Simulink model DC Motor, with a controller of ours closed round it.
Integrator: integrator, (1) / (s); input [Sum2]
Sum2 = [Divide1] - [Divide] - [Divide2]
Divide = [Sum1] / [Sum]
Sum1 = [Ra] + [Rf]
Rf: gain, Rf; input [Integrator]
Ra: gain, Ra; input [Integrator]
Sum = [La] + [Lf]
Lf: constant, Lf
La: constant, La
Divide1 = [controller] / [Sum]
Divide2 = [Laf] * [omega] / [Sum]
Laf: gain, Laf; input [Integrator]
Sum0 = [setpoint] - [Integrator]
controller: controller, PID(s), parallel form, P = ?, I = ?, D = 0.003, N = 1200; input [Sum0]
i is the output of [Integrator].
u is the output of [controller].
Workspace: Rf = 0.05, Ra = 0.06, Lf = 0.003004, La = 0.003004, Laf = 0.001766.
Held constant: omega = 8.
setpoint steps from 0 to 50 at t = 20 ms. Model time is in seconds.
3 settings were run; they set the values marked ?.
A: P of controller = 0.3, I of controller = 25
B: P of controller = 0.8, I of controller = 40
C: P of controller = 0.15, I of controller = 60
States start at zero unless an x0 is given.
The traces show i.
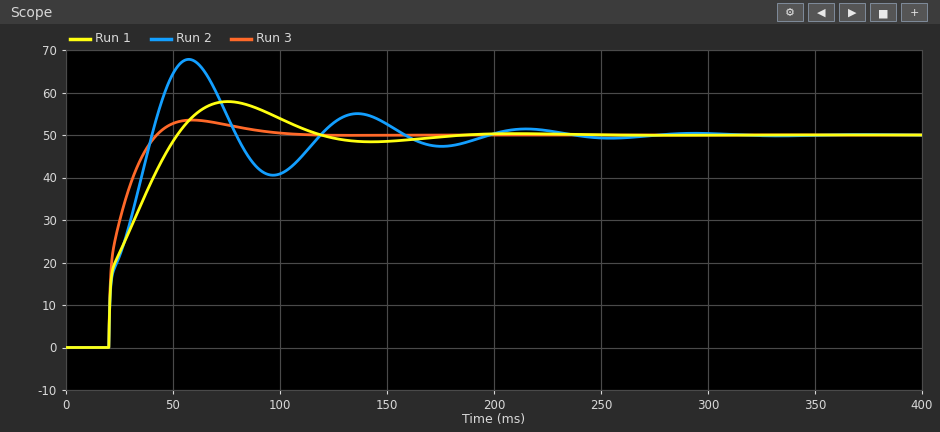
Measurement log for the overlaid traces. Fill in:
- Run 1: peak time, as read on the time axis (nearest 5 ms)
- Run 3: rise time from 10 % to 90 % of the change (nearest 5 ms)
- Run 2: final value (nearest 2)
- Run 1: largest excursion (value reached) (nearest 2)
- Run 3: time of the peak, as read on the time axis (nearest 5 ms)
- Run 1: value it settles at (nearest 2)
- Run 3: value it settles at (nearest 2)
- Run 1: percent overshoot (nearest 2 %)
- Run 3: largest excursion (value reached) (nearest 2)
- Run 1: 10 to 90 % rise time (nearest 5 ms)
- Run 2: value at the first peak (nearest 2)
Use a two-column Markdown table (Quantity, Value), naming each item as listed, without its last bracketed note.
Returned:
| Quantity | Value |
|---|---|
| Run 1: peak time, as read on the time axis | 75 ms |
| Run 3: rise time from 10 % to 90 % of the change | 15 ms |
| Run 2: final value | 50 |
| Run 1: largest excursion (value reached) | 58 |
| Run 3: time of the peak, as read on the time axis | 60 ms |
| Run 1: value it settles at | 50 |
| Run 3: value it settles at | 50 |
| Run 1: percent overshoot | 16 % |
| Run 3: largest excursion (value reached) | 54 |
| Run 1: 10 to 90 % rise time | 25 ms |
| Run 2: value at the first peak | 68 |
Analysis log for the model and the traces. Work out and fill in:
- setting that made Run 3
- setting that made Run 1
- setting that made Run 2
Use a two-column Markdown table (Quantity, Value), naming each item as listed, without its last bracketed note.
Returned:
| Quantity | Value |
|---|---|
| setting that made Run 3 | B |
| setting that made Run 1 | A |
| setting that made Run 2 | C |
